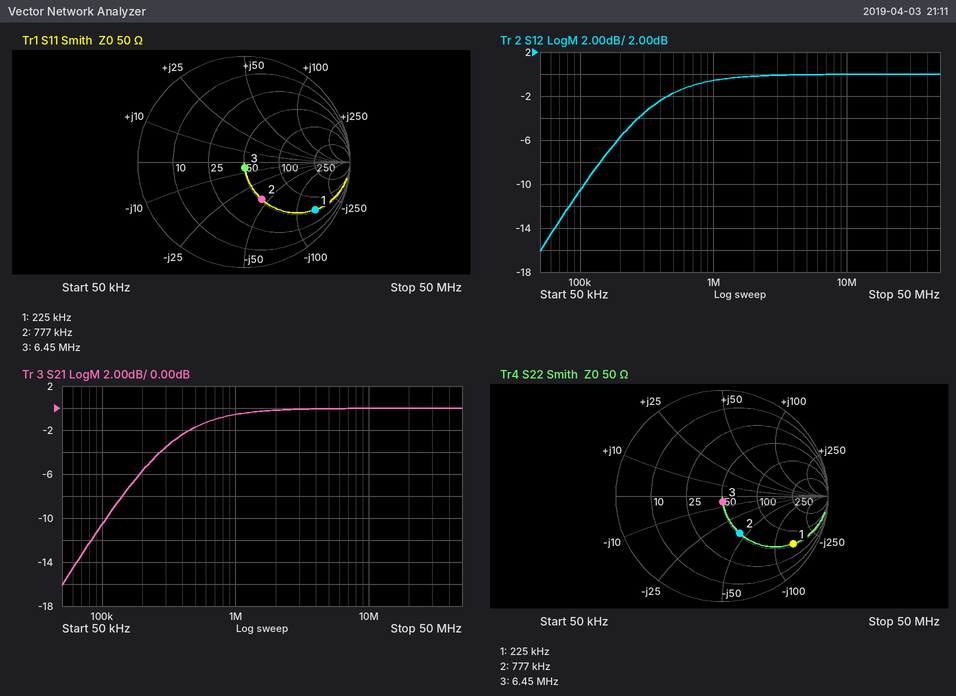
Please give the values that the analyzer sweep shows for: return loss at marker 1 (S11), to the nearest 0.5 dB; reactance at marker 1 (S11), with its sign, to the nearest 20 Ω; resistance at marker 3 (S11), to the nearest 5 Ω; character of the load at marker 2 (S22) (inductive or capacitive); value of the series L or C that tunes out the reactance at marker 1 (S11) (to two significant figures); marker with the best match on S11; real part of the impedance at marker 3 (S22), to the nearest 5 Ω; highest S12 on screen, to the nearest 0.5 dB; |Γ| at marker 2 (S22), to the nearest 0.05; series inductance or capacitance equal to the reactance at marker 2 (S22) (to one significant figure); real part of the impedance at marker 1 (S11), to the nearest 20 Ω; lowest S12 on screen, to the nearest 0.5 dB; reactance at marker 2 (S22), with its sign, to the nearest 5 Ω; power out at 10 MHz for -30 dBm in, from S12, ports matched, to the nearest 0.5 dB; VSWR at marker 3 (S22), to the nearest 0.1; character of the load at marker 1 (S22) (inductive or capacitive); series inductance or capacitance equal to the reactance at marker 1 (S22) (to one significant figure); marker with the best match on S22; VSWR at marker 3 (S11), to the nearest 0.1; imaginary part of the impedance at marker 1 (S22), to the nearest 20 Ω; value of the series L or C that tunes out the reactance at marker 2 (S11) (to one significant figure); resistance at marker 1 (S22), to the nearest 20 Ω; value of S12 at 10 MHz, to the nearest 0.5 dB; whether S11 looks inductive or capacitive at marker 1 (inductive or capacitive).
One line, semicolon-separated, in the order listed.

2.0 dB; -140 Ω; 50 Ω; capacitive; 100 µH; marker 3; 50 Ω; 0.0 dB; 0.40; 5 nF; 60 Ω; -16.0 dB; -45 Ω; -30.0 dBm; 1.1; capacitive; 5 nF; marker 3; 1.1; -140 Ω; 9 µH; 60 Ω; 0.0 dB; capacitive
